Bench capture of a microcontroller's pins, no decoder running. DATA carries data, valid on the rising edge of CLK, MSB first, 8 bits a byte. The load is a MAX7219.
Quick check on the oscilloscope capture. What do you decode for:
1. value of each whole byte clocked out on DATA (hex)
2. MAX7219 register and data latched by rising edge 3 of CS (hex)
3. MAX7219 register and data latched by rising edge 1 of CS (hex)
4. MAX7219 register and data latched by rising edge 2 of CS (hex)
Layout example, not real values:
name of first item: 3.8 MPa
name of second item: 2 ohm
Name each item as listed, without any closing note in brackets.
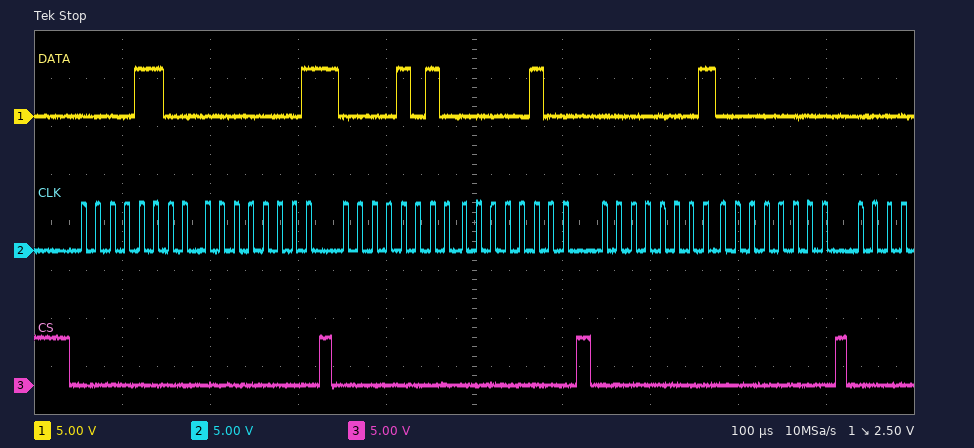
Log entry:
value of each whole byte clocked out on DATA: 0x0C 0x01 0x0A 0x04 0x01 0x00
MAX7219 register and data latched by rising edge 3 of CS: register 0x1, data 0x00
MAX7219 register and data latched by rising edge 1 of CS: register 0xC, data 0x01
MAX7219 register and data latched by rising edge 2 of CS: register 0xA, data 0x04
